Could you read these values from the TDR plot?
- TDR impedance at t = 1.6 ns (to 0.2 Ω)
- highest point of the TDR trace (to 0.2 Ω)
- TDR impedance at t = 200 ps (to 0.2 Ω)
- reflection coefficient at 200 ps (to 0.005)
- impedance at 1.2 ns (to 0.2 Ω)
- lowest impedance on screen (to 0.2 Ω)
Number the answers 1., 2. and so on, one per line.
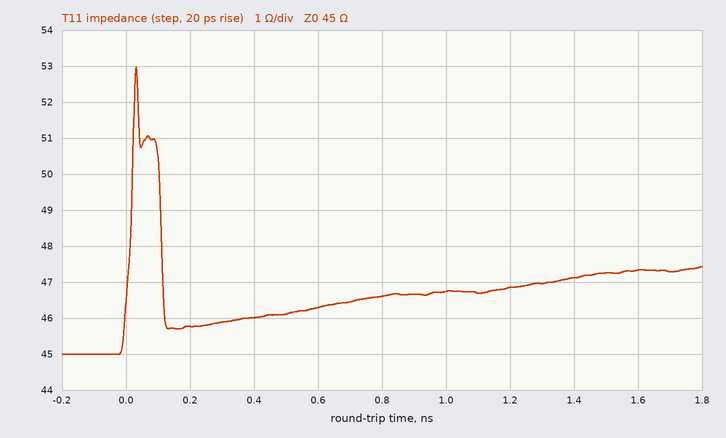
1. 47.4 Ω
2. 53.0 Ω
3. 45.8 Ω
4. +0.010
5. 46.8 Ω
6. 45.0 Ω
